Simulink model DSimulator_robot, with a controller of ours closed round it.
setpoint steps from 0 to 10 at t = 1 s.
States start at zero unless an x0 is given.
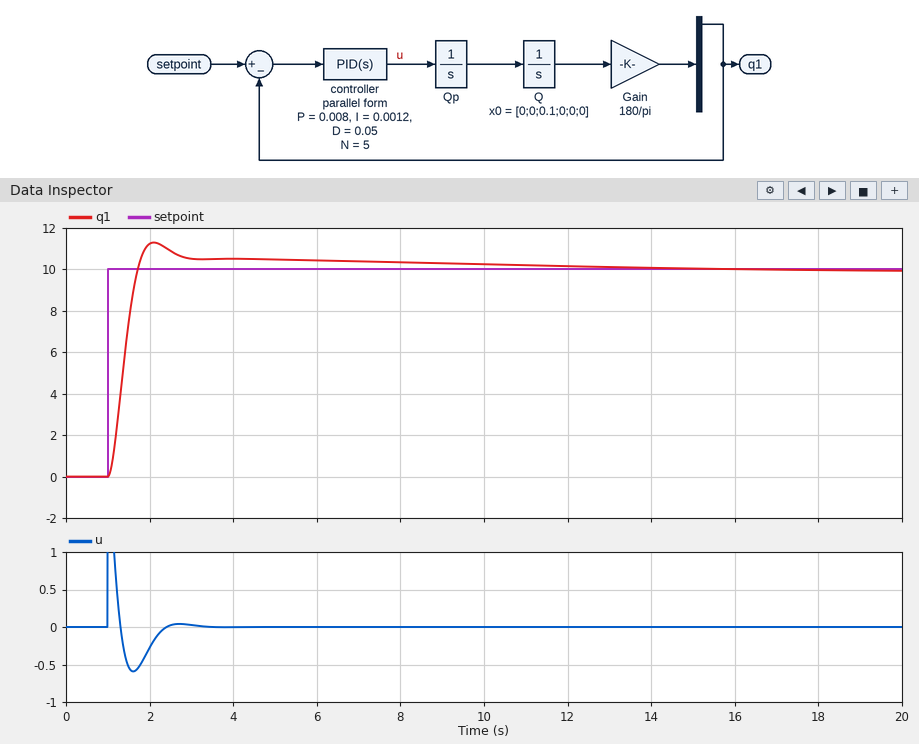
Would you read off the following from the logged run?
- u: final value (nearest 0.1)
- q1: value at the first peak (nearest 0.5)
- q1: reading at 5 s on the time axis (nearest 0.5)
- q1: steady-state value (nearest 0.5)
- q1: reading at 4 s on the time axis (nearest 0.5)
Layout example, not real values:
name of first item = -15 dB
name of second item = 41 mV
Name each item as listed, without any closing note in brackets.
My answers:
u: final value = 0.0
q1: value at the first peak = 11.5
q1: reading at 5 s on the time axis = 10.5
q1: steady-state value = 10.0
q1: reading at 4 s on the time axis = 10.5
